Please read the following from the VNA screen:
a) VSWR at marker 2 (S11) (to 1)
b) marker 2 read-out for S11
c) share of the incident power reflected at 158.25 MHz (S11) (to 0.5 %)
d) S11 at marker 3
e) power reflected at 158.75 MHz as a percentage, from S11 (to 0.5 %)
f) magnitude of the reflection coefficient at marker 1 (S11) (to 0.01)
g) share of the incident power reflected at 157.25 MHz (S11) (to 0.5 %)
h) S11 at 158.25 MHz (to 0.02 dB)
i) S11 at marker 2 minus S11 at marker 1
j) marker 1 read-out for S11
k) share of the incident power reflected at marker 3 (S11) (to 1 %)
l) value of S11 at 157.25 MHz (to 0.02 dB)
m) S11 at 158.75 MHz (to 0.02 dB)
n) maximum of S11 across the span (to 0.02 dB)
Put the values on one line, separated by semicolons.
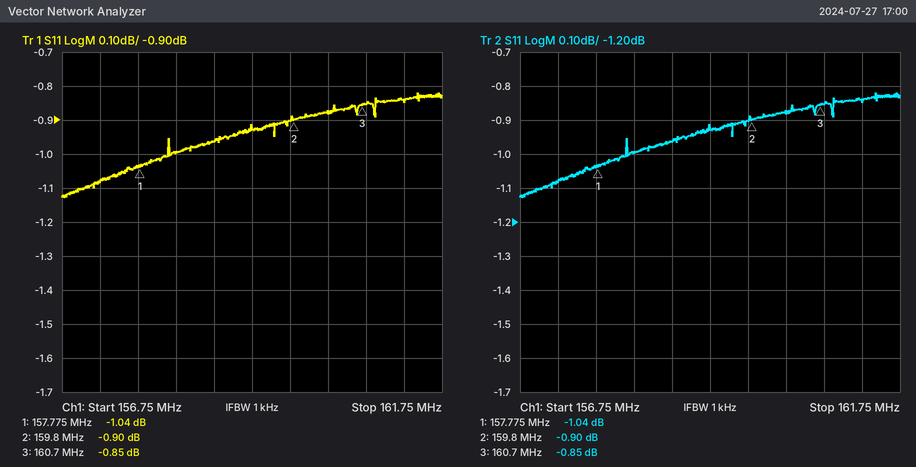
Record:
19; -0.90 dB; 79.5 %; -0.85 dB; 80.0 %; 0.89; 78.0 %; -1.00 dB; 0.14 dB; -1.04 dB; 82 %; -1.08 dB; -0.96 dB; -0.82 dB
